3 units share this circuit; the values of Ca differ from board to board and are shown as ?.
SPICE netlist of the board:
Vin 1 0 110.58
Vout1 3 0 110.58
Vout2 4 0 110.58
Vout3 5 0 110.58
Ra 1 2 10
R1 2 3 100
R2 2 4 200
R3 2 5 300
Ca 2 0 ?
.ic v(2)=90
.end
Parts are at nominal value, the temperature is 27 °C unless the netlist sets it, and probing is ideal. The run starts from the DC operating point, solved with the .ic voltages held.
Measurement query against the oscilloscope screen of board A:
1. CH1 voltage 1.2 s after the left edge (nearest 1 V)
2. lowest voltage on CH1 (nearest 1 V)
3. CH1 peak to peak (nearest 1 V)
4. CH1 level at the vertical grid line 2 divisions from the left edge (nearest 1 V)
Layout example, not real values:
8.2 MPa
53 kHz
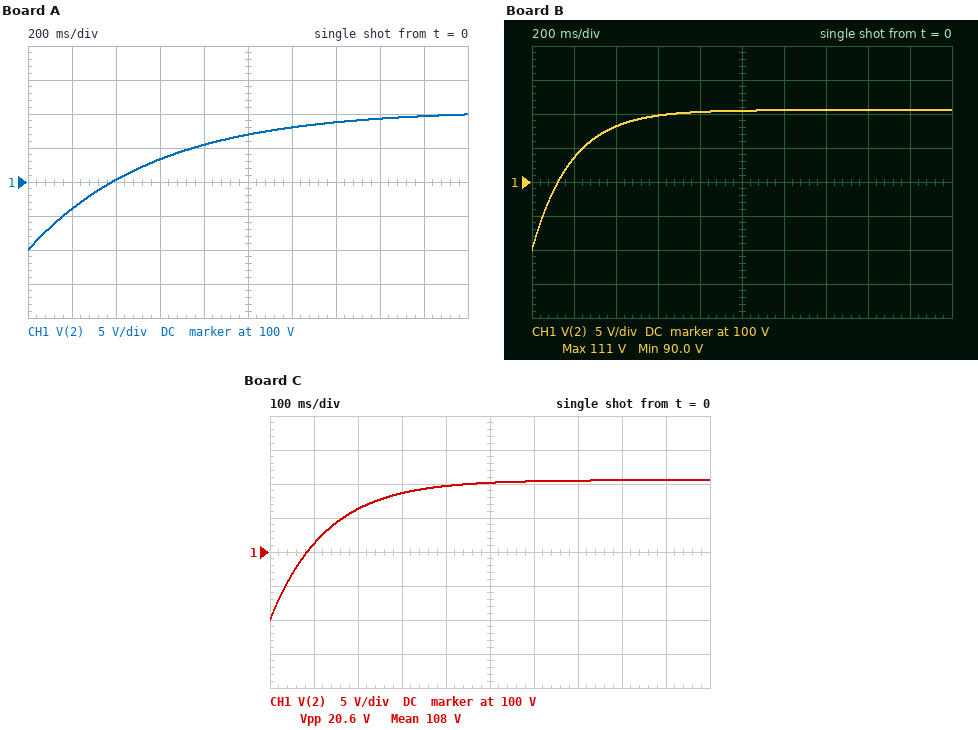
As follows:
108 V
90 V
20 V
100 V
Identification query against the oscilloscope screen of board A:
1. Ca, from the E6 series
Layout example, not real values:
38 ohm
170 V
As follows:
68 mF
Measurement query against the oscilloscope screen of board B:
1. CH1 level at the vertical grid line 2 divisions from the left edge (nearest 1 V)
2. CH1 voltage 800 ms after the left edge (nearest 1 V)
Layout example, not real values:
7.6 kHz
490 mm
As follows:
108 V
110 V
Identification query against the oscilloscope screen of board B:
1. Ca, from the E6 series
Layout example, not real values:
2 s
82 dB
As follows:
22 mF
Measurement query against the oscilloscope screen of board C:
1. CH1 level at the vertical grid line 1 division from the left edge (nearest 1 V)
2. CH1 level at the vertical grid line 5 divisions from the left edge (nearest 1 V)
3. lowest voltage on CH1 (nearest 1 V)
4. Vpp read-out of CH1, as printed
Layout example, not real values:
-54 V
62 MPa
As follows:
101 V
110 V
90 V
20.6 V
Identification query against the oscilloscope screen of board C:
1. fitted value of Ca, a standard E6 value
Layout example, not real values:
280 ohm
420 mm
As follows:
15 mF
